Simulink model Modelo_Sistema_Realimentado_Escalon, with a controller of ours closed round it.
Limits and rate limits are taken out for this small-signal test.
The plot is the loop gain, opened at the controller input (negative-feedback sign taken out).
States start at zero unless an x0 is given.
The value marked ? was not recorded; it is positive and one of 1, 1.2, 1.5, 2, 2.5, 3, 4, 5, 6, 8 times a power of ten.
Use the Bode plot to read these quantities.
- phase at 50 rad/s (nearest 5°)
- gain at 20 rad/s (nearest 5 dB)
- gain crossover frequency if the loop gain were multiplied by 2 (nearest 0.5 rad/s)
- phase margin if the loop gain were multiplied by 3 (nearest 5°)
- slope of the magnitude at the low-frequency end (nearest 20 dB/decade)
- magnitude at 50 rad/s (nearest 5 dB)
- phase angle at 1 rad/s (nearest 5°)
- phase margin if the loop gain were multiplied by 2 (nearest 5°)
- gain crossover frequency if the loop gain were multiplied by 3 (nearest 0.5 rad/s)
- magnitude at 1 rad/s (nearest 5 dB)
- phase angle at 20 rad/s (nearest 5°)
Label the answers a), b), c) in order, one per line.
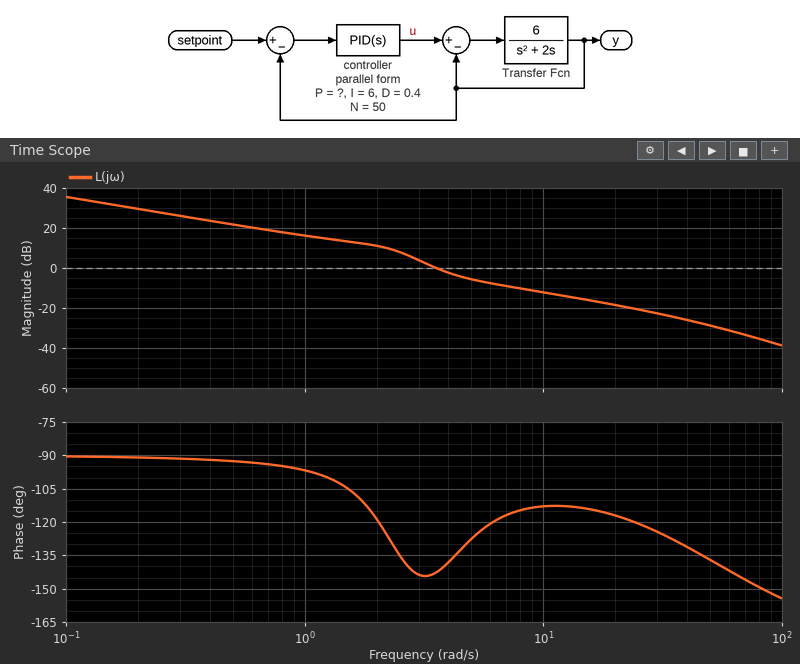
a) -135°
b) -20 dB
c) 5.0 rad/s
d) 65°
e) -20 dB/decade
f) -30 dB
g) -95°
h) 55°
i) 7.5 rad/s
j) 15 dB
k) -115°
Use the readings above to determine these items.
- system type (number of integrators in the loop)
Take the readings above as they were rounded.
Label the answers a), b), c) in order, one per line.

a) 1
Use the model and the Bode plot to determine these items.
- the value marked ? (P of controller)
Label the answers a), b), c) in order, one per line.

a) 1.5
